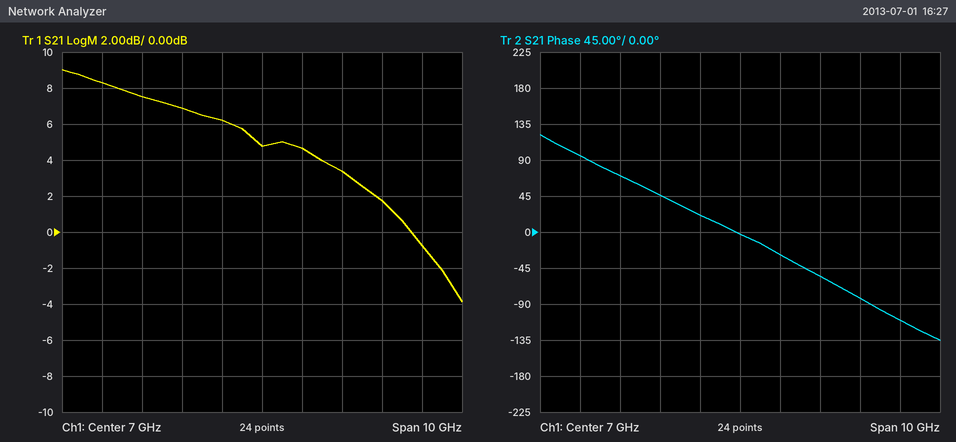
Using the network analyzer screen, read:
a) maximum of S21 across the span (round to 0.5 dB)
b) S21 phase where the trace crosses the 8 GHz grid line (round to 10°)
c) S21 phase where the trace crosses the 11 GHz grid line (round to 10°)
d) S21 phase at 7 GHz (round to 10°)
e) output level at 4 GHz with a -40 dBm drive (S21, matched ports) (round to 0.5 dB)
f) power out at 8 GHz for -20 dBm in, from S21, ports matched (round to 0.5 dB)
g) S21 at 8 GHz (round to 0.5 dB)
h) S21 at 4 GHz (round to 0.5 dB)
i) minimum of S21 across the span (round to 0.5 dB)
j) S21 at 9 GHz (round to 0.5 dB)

9.0 dB
-30°
-110°
0°
-32.5 dBm
-15.5 dBm
4.5 dB
7.5 dB
-4.0 dB
3.5 dB
